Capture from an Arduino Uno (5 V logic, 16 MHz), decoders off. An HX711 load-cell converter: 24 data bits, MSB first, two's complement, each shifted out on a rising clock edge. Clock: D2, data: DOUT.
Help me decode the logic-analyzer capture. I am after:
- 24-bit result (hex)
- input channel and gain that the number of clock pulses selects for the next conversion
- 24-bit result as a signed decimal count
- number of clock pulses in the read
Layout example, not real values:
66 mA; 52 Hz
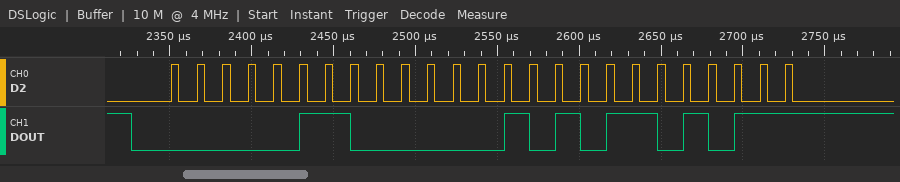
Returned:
0x06056B; channel A, gain 128; 394603; 25
